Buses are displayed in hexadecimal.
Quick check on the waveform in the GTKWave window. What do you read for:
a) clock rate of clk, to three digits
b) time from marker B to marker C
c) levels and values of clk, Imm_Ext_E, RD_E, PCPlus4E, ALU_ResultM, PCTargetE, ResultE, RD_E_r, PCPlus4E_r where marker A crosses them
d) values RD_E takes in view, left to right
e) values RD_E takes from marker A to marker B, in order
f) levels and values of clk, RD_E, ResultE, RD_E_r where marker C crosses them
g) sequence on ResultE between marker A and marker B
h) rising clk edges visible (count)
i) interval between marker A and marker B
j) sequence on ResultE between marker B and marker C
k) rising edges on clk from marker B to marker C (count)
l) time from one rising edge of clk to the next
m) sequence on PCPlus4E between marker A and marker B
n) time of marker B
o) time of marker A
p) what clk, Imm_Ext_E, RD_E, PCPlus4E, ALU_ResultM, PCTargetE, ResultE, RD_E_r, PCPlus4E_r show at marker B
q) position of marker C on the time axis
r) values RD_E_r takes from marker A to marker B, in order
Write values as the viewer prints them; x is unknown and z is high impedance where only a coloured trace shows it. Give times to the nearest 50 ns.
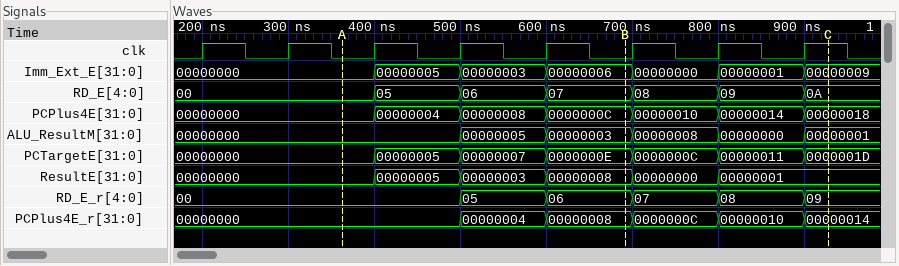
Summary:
10.0 MHz
250 ns
clk=0, Imm_Ext_E=00000000, RD_E=00, PCPlus4E=00000000, ALU_ResultM=00000000, PCTargetE=00000000, ResultE=00000000, RD_E_r=00, PCPlus4E_r=00000000
00, 05, 06, 07, 08, 09, 0A
00, 05, 06, 07
clk=1, RD_E=0A, ResultE=00000001, RD_E_r=09
00000000, 00000005, 00000003, 00000008
8
350 ns
00000008, 00000000, 00000001
3
100 ns
00000000, 00000004, 00000008, 0000000C
700 ns
350 ns
clk=0, Imm_Ext_E=00000006, RD_E=07, PCPlus4E=0000000C, ALU_ResultM=00000003, PCTargetE=0000000E, ResultE=00000008, RD_E_r=06, PCPlus4E_r=00000008
950 ns
00, 05, 06
